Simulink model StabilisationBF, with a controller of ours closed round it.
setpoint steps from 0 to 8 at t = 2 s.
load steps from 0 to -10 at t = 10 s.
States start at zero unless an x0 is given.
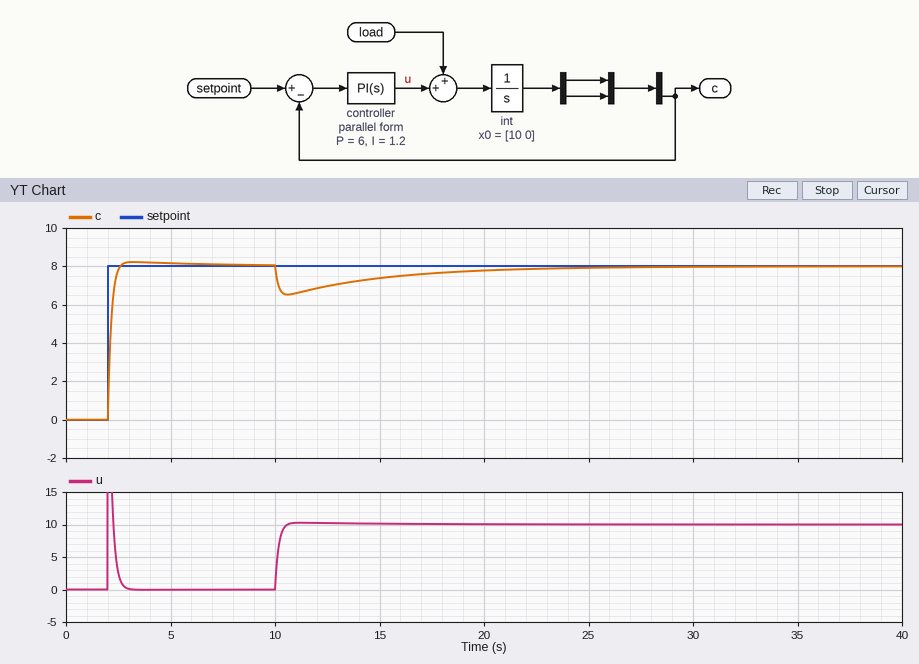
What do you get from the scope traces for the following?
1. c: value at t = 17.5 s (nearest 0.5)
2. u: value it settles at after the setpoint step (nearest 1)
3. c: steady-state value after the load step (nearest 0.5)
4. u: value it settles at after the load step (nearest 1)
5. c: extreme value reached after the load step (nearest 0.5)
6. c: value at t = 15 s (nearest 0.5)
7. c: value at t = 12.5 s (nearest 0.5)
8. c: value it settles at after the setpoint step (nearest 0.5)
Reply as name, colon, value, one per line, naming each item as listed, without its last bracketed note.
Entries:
c: value at t = 17.5 s: 7.5
u: value it settles at after the setpoint step: 0
c: steady-state value after the load step: 8.0
u: value it settles at after the load step: 10
c: extreme value reached after the load step: 6.5
c: value at t = 15 s: 7.5
c: value at t = 12.5 s: 7.0
c: value it settles at after the setpoint step: 8.0
